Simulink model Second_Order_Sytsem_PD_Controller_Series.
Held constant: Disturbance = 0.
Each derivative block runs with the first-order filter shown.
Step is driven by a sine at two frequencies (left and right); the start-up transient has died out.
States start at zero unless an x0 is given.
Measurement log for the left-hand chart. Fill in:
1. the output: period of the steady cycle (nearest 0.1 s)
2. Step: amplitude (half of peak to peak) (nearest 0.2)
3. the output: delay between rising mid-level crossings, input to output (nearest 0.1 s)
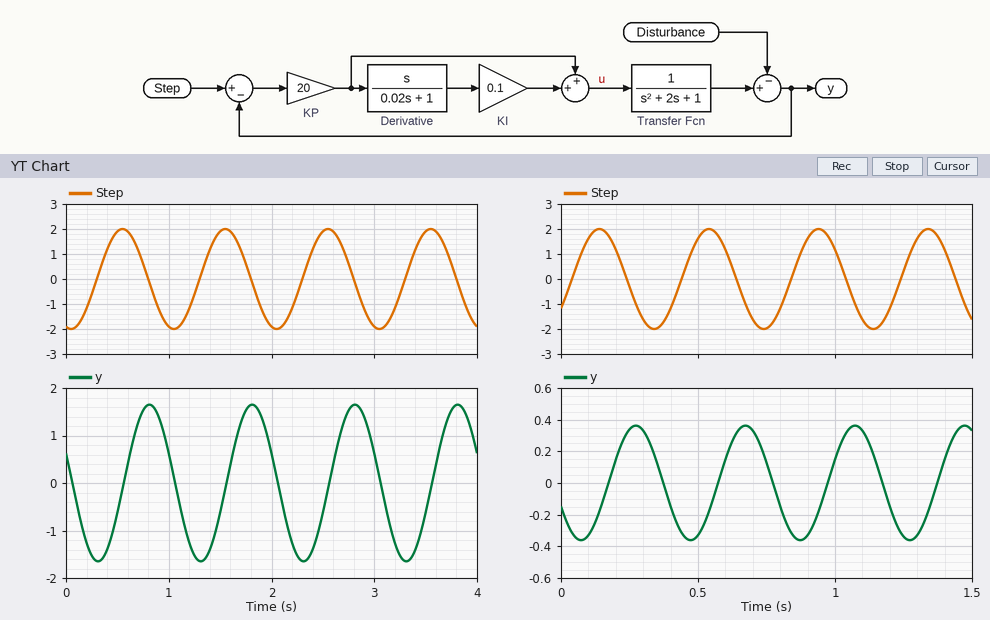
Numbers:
1.0 s
2.0
0.3 s
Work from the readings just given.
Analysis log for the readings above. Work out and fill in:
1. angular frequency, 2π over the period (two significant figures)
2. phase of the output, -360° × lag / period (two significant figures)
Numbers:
6.3 rad/s
-110°
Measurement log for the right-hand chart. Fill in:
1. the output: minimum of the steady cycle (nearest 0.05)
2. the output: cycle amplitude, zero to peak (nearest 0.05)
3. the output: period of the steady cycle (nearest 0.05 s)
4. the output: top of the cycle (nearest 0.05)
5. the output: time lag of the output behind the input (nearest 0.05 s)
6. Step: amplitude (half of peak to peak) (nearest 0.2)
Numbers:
-0.35
0.35
0.40 s
0.35
0.15 s
2.0
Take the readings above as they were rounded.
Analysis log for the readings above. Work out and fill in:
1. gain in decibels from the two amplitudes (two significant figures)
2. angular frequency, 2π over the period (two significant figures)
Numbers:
-15 dB
16 rad/s
